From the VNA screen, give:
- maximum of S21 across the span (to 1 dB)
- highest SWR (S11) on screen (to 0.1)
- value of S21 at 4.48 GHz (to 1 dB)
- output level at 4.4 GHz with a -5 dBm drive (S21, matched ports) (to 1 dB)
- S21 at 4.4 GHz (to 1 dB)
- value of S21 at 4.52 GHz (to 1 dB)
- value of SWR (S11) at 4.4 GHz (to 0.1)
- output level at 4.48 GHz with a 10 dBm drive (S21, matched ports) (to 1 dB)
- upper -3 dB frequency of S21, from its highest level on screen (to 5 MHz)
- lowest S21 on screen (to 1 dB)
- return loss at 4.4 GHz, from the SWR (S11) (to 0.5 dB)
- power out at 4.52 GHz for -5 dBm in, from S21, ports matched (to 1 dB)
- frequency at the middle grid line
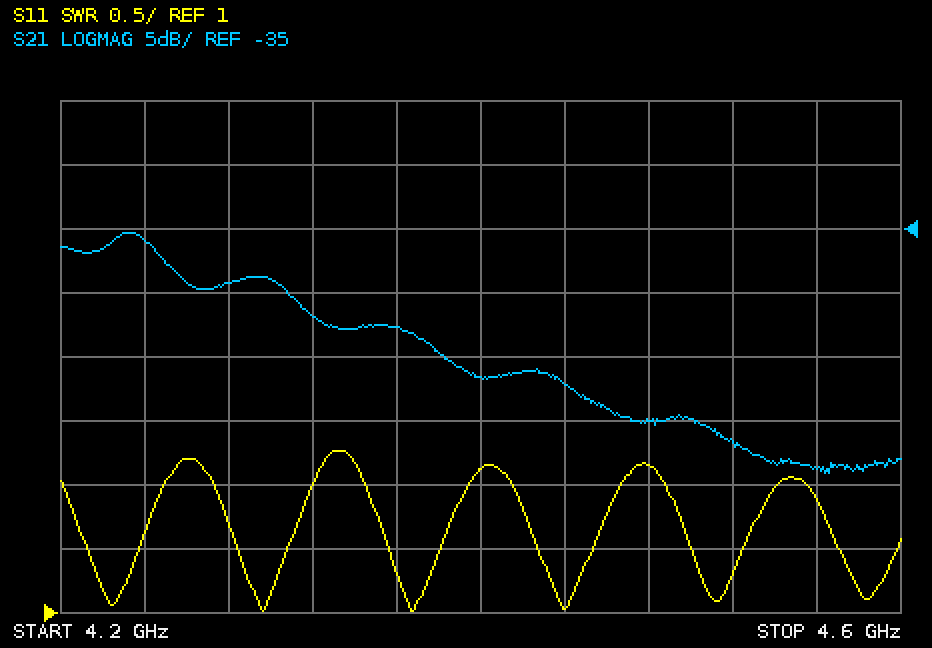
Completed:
-35 dB
2.3
-50 dB
-52 dBm
-47 dB
-52 dB
2.1
-40 dBm
4.255 GHz
-54 dB
9.0 dB
-57 dBm
4.4 GHz
